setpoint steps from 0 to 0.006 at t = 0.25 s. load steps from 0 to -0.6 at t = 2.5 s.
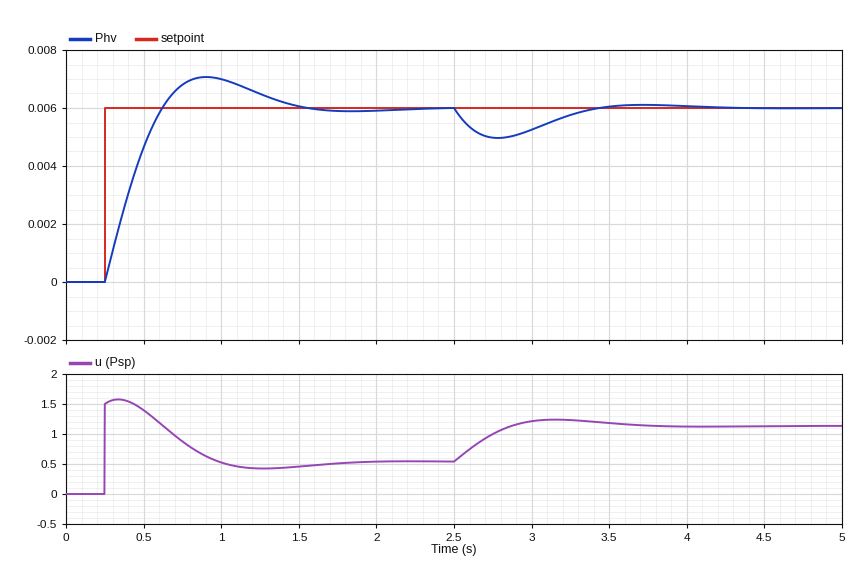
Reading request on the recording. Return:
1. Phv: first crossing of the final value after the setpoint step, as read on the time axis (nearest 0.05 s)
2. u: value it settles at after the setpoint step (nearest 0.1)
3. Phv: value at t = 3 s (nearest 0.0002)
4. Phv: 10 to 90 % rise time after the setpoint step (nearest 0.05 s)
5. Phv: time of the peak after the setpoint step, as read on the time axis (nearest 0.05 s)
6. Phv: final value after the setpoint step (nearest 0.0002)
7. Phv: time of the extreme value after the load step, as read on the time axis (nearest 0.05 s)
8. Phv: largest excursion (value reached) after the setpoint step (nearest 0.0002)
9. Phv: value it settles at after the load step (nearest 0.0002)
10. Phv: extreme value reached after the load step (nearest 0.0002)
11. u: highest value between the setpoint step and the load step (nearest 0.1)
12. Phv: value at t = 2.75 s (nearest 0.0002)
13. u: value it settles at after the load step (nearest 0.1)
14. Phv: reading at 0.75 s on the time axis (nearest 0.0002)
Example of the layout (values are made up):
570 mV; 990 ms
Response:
0.60 s; 0.5; 0.0052; 0.30 s; 0.90 s; 0.0060; 2.80 s; 0.0070; 0.0060; 0.0050; 1.6; 0.0050; 1.1; 0.0068
